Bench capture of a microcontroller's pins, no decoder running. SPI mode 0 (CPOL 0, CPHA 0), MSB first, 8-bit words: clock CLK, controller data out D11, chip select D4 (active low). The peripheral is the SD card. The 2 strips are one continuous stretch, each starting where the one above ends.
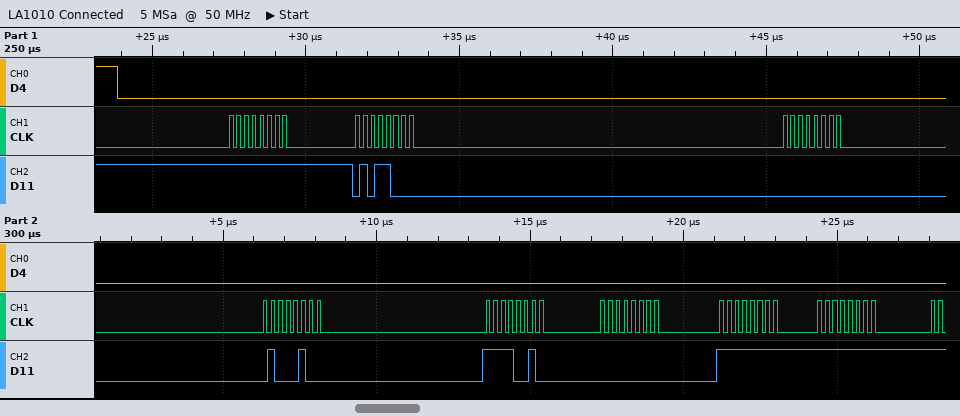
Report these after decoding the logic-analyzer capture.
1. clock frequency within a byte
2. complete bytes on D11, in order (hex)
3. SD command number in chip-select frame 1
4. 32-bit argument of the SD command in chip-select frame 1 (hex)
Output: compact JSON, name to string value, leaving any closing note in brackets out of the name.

{"clock frequency within a byte": "4 MHz", "complete bytes on D11, in order": "FF 58 00 44 F2 00 FF FF", "SD command number in chip-select frame 1": "CMD24", "32-bit argument of the SD command in chip-select frame 1": "0x0044F200"}
